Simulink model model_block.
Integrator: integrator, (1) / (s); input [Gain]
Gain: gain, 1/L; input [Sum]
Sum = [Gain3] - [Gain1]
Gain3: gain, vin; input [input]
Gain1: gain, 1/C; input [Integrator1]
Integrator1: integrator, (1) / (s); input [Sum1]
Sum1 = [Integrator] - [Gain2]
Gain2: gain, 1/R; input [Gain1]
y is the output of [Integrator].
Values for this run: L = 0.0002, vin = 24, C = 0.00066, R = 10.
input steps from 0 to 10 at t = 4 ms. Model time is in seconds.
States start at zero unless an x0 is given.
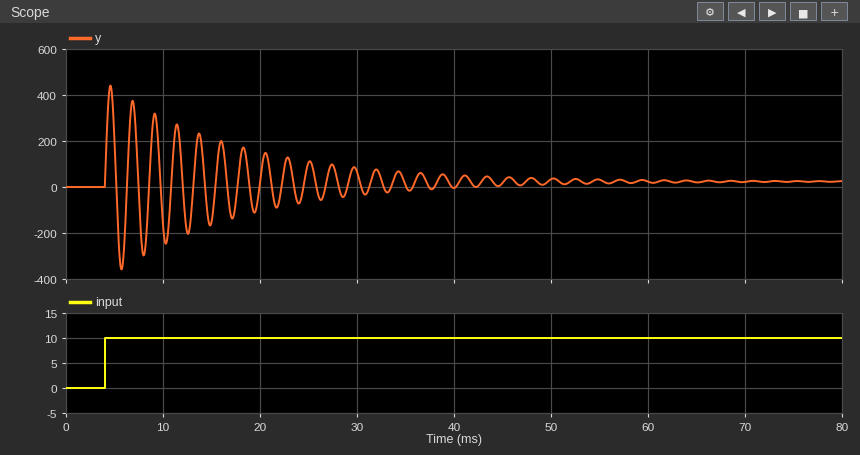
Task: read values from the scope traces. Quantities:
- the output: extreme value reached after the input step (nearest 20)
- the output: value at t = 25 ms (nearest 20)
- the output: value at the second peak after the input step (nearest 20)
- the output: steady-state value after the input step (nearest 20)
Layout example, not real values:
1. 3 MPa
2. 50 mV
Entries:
1. 440
2. 100
3. 380
4. 20
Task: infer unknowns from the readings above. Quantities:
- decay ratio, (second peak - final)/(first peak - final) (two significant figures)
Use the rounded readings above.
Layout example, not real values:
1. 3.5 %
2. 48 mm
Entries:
1. 0.86
